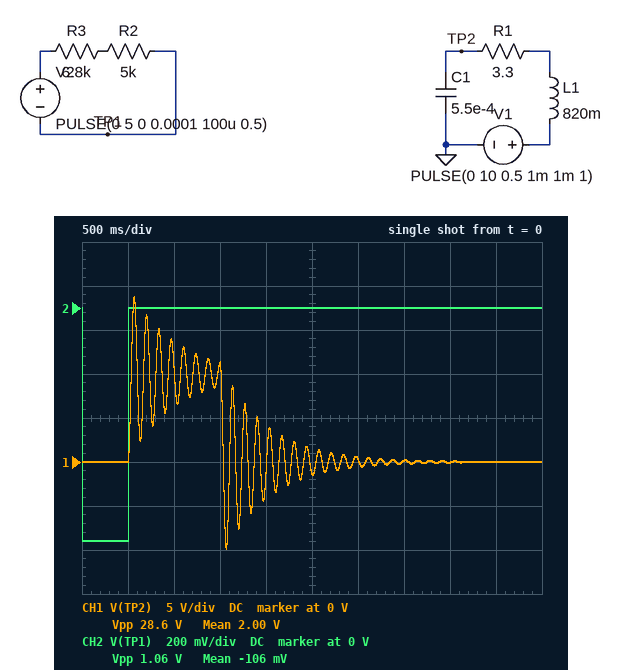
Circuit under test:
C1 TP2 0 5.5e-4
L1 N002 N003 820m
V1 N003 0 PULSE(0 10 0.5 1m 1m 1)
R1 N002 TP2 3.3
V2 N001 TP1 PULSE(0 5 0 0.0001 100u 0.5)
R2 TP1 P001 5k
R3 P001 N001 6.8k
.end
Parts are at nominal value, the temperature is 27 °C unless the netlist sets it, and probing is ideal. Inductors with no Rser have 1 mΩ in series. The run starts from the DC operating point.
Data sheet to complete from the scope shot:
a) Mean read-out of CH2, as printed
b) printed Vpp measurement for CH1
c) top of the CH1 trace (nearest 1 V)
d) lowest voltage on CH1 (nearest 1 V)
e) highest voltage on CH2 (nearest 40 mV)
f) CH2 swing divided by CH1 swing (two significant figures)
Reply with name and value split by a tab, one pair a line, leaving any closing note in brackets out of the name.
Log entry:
Mean read-out of CH2, as printed	-106 mV
printed Vpp measurement for CH1	28.6 V
top of the CH1 trace	19 V
lowest voltage on CH1	-10 V
highest voltage on CH2	0 V
CH2 swing divided by CH1 swing	0.037
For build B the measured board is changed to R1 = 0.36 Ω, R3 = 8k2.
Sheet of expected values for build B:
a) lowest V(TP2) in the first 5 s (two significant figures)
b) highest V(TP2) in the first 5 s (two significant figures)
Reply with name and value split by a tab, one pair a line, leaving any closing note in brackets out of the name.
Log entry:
lowest V(TP2) in the first 5 s	-18 V
highest V(TP2) in the first 5 s	20 V
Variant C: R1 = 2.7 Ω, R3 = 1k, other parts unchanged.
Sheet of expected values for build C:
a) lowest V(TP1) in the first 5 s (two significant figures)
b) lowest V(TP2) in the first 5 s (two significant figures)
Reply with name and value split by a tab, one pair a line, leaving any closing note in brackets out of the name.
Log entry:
lowest V(TP1) in the first 5 s	-2.1 V
lowest V(TP2) in the first 5 s	-11 V
